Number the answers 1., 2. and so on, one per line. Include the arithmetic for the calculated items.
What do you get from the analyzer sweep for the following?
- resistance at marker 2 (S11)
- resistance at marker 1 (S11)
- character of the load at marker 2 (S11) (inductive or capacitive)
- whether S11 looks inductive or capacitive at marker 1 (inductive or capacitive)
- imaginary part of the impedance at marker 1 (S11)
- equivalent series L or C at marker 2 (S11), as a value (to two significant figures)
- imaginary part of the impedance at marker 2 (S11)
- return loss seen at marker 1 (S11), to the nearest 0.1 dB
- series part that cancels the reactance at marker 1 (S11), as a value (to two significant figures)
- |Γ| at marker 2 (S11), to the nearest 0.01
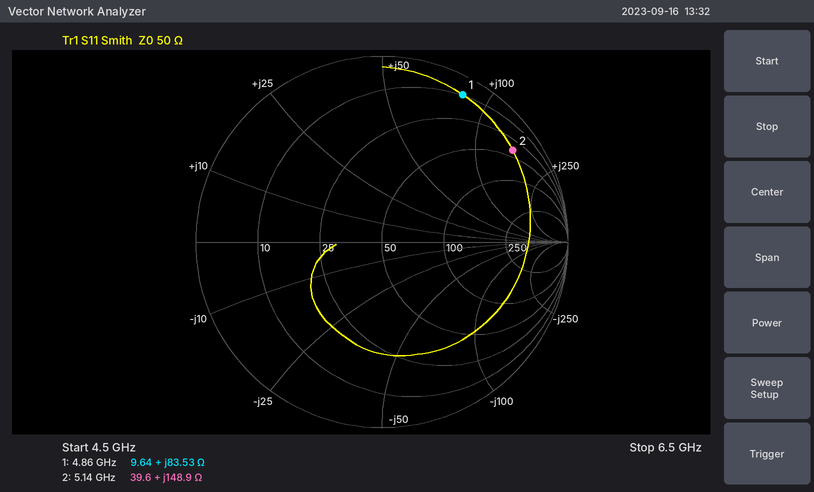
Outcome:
1. 39.6 Ω
2. 9.64 Ω
3. inductive
4. inductive
5. +83.53 Ω
6. L = 148.9 Ω/(2π × 5.14 GHz) ≈ 4.6 nH
7. +148.9 Ω
8. 0.9 dB
9. C = 1/(2π × 4.86 GHz × 83.53 Ω) ≈ 392 fF, so 390 fF to two significant figures
10. 0.86
